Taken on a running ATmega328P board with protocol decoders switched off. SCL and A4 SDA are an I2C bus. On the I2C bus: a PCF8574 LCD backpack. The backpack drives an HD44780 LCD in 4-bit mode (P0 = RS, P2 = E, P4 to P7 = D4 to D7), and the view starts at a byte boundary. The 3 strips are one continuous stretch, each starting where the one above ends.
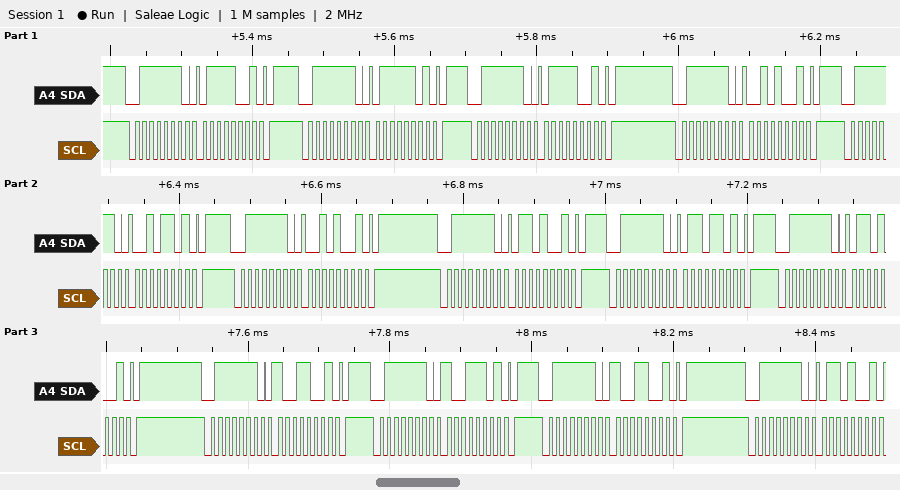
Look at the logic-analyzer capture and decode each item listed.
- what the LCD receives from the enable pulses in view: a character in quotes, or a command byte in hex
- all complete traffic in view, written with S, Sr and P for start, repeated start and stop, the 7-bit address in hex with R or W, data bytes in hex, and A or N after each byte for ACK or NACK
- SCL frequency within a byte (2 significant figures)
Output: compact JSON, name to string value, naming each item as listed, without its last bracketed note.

{"what the LCD receives from the enable pulses in view: a character in quotes, or a command byte in hex": "'r' 'i'", "all complete traffic in view, written with S, Sr and P for start, repeated start and stop, the 7-bit address in hex with R or W, data bytes in hex, and A or N after each byte for ACK or NACK": "S 3FW A 79 A P S 3FW A 7D A P S 3FW A 79 A P S 3FW A 29 A P S 3FW A 2D A P S 3FW A 29 A P S 3FW A 69 A P S 3FW A 6D A P S 3FW A 69 A P S 3FW A 99 A P S 3FW A 9D A P S 3FW A 99 A P S 3FW A 69 A", "SCL frequency within a byte": "100 kHz"}
